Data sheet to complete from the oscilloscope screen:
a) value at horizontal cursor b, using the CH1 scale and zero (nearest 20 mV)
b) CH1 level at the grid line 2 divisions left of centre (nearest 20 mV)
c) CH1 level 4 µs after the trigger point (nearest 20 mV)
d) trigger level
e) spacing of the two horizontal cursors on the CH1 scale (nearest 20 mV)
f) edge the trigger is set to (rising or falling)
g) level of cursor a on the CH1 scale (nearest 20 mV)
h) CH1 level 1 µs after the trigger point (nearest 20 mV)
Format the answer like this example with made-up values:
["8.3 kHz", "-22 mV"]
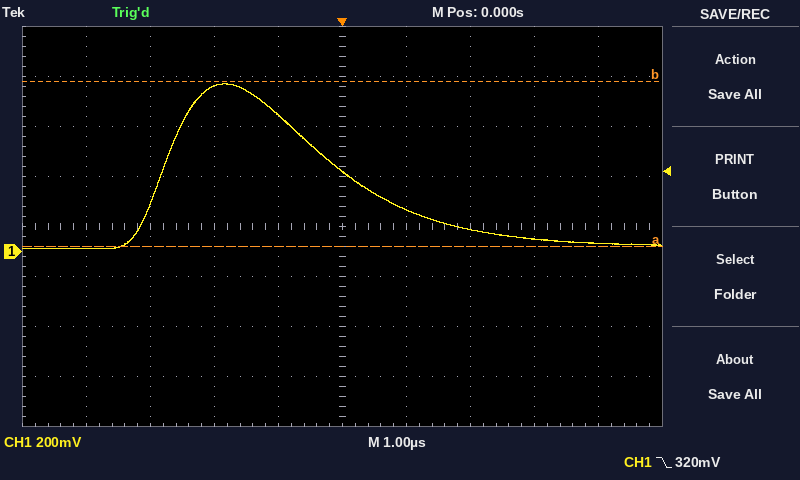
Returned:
["680 mV", "660 mV", "40 mV", "320 mV", "660 mV", "falling", "20 mV", "160 mV"]
